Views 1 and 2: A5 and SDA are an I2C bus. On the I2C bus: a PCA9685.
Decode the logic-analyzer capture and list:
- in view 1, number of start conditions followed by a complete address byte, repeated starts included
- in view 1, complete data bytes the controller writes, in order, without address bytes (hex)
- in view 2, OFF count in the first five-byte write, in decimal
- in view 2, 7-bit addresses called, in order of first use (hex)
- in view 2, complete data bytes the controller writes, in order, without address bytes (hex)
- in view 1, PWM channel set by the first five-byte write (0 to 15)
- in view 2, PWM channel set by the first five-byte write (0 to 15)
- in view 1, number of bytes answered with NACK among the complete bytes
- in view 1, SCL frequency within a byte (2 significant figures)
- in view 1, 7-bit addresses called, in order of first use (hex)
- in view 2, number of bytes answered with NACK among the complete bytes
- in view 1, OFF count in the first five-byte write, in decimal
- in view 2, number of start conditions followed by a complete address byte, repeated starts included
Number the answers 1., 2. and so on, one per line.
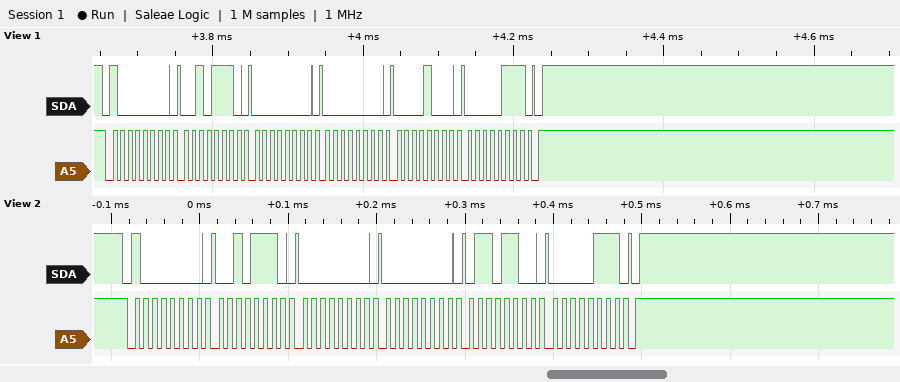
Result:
1. 1
2. 2E 00 00 08 07
3. 1900
4. 0x40
5. 2E 00 00 6C 07
6. 10
7. 10
8. 0
9. 100 kHz
10. 0x40
11. 0
12. 1800
13. 1
